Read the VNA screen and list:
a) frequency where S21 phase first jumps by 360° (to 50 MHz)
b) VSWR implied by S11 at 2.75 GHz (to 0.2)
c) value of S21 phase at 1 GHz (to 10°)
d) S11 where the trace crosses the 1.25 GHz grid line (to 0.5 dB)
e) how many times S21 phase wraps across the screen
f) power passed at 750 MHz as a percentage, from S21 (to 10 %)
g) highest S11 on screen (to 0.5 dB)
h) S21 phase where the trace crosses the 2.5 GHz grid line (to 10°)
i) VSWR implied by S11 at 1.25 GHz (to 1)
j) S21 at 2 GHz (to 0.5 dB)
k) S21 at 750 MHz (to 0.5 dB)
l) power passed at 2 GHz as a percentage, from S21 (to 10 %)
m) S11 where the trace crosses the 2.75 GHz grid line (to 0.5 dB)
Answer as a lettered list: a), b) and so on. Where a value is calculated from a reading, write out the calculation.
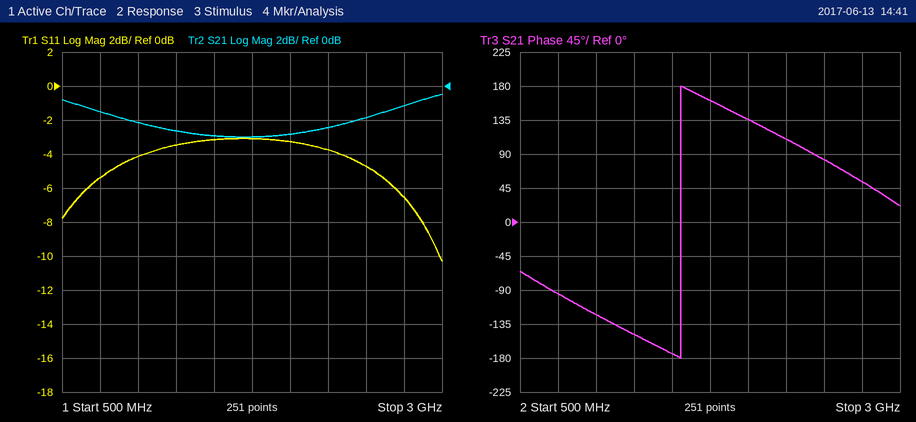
a) 1.55 GHz
b) |Γ| = 10^(-6.5/20) = 0.4732; VSWR = (1 + 0.4732)/(1 − 0.4732) ≈ 2.8
c) -120°
d) -3.5 dB
e) 1
f) 10^(-1.5/10) ≈ 70.8 %, so 70 % to the nearest 10 %
g) -3.0 dB
h) 80°
i) |Γ| = 10^(-3.5/20) = 0.6683; VSWR = (1 + 0.6683)/(1 − 0.6683) ≈ 5
j) -3.0 dB
k) -1.5 dB
l) 10^(-3/10) ≈ 50 %
m) -6.5 dB
